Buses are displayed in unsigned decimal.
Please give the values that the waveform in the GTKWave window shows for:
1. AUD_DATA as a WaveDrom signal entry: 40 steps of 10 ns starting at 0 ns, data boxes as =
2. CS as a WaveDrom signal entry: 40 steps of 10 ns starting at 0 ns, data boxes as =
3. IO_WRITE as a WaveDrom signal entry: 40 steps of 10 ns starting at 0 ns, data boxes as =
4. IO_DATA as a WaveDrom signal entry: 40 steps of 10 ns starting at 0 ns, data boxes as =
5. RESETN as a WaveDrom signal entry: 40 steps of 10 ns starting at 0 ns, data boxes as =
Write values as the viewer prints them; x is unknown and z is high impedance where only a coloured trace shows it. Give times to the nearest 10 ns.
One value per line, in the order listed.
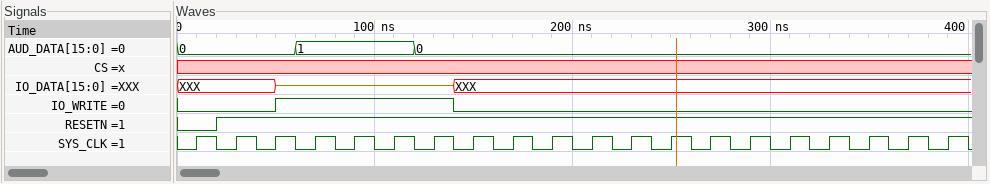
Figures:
{name: 'AUD_DATA', wave: '=.....=.....=...........................', data: '0 1 0'}
{name: 'CS', wave: 'x.......................................'}
{name: 'IO_WRITE', wave: '0....1........0.........................'}
{name: 'IO_DATA', wave: 'x....z........x.........................'}
{name: 'RESETN', wave: '0.1.....................................'}
